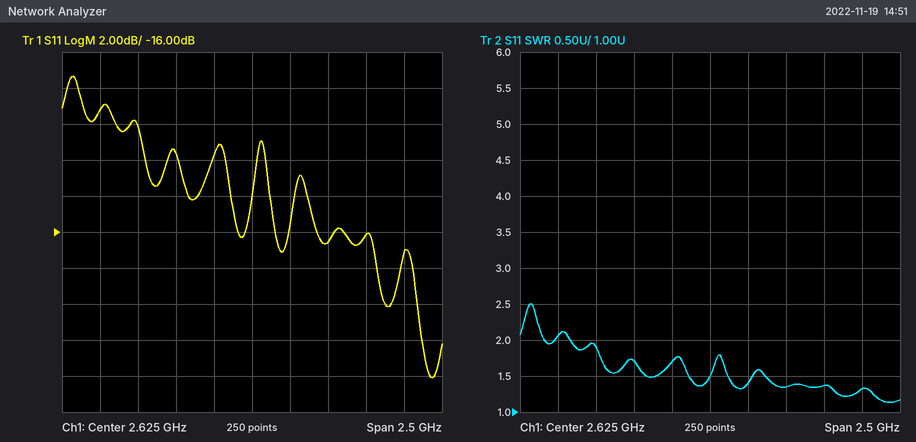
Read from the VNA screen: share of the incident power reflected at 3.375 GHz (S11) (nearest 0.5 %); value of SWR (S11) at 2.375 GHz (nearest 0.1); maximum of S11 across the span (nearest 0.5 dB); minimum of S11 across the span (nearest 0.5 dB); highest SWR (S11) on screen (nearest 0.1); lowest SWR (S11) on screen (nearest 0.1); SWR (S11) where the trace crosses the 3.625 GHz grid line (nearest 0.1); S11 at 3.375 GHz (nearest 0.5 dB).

2.5 %
1.7
-7.5 dB
-24.0 dB
2.5
1.1
1.3
-16.0 dB
